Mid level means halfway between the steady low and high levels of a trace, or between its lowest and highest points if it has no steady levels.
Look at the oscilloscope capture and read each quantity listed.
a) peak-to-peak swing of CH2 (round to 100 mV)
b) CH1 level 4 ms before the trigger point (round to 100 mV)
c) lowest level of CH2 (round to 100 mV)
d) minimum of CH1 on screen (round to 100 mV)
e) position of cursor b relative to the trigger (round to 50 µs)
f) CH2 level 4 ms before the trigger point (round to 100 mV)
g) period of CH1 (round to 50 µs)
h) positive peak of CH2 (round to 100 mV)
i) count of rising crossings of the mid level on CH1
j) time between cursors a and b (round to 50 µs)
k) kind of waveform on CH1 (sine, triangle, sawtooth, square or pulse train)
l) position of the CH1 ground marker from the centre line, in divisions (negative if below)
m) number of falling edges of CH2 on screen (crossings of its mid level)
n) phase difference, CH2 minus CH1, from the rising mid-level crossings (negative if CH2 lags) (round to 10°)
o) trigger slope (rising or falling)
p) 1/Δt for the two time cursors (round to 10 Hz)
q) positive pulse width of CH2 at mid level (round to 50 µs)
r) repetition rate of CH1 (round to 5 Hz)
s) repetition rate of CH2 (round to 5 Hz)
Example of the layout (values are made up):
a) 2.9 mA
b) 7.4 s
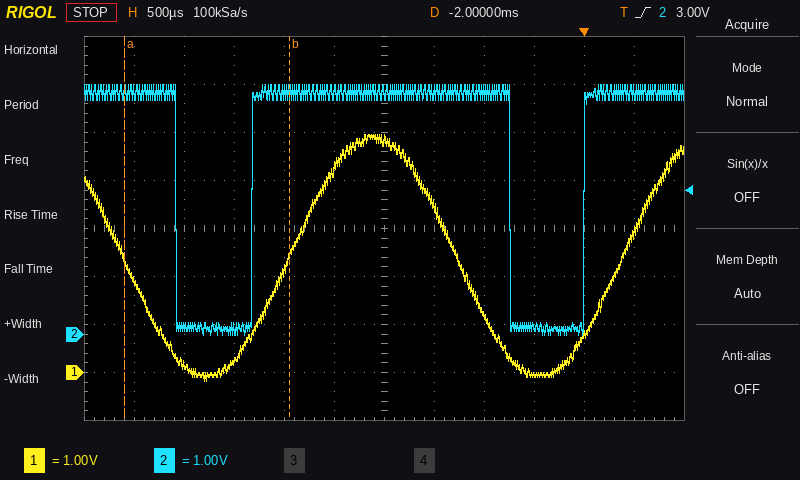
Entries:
a) 5.2 V
b) 200 mV
c) 0.0 V
d) -200 mV
e) -2.95 ms
f) 200 mV
g) 3.35 ms
h) 5.2 V
i) 2
j) 1.65 ms
k) sine
l) -3.0 div
m) 2
n) +40°
o) rising
p) 610 Hz
q) 2.60 ms
r) 300 Hz
s) 300 Hz
